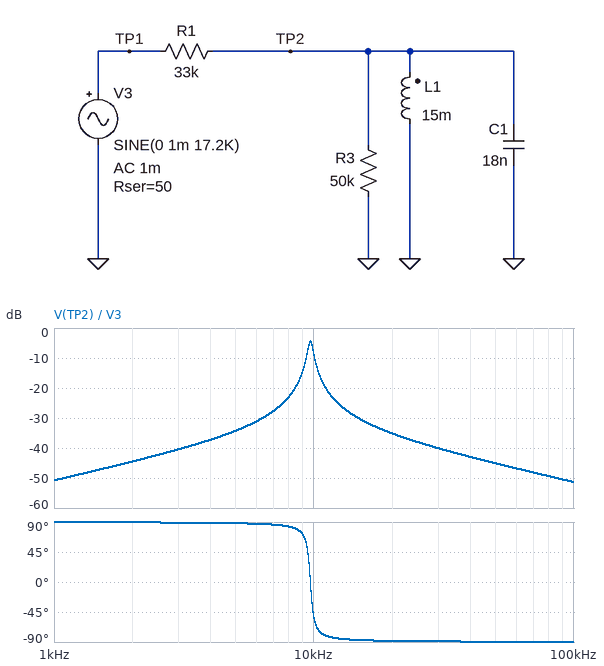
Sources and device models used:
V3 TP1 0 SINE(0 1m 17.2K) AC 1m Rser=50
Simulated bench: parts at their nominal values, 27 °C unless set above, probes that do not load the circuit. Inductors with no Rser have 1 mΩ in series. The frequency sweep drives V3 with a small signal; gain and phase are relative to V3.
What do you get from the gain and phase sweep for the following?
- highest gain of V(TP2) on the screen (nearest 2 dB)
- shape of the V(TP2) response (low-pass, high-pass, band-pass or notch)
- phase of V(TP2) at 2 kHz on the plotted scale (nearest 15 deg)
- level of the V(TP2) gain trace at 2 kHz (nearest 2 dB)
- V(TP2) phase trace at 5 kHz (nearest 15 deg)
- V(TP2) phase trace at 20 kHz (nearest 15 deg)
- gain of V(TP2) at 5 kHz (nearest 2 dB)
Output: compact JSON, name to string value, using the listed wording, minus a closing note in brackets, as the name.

{"highest gain of V(TP2) on the screen": "-4 dB", "shape of the V(TP2) response": "band-pass", "phase of V(TP2) at 2 kHz on the plotted scale": "90 deg", "level of the V(TP2) gain trace at 2 kHz": "-44 dB", "V(TP2) phase trace at 5 kHz": "90 deg", "V(TP2) phase trace at 20 kHz": "-90 deg", "gain of V(TP2) at 5 kHz": "-34 dB"}
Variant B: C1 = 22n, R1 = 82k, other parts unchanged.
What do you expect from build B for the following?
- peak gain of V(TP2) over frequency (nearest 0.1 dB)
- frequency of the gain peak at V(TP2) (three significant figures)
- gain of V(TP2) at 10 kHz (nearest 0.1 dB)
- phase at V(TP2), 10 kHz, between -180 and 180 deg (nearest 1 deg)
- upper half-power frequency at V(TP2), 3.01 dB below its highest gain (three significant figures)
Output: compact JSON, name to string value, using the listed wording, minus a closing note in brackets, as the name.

{"peak gain of V(TP2) over frequency": "-8.4 dB", "frequency of the gain peak at V(TP2)": "8.76 kHz", "gain of V(TP2) at 10 kHz": "-28.5 dB", "phase at V(TP2), 10 kHz, between -180 and 180 deg": "-84 deg", "upper half-power frequency at V(TP2), 3.01 dB below its highest gain": "8.88 kHz"}
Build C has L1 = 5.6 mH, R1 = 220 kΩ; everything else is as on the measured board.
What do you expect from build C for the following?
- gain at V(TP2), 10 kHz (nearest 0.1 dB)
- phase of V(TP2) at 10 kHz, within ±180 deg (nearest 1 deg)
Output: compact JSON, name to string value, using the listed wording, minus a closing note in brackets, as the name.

{"gain at V(TP2), 10 kHz": "-51.5 dB", "phase of V(TP2) at 10 kHz, within ±180 deg": "89 deg"}
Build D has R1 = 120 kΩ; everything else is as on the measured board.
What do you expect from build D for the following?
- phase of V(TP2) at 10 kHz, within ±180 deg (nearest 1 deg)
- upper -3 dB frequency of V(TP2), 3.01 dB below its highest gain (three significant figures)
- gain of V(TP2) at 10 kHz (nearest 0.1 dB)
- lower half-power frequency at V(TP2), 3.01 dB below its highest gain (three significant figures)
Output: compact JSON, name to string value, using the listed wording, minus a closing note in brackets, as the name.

{"phase of V(TP2) at 10 kHz, within ±180 deg": "-68 deg", "upper -3 dB frequency of V(TP2), 3.01 dB below its highest gain": "9.81 kHz", "gain of V(TP2) at 10 kHz": "-19.1 dB", "lower half-power frequency at V(TP2), 3.01 dB below its highest gain": "9.56 kHz"}
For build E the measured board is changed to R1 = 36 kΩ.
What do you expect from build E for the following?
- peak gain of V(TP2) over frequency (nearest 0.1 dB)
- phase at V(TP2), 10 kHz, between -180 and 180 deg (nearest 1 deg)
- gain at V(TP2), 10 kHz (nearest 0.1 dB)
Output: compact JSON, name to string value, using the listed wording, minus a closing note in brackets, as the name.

{"peak gain of V(TP2) over frequency": "-4.7 dB", "phase at V(TP2), 10 kHz, between -180 and 180 deg": "-56 deg", "gain at V(TP2), 10 kHz": "-9.7 dB"}
